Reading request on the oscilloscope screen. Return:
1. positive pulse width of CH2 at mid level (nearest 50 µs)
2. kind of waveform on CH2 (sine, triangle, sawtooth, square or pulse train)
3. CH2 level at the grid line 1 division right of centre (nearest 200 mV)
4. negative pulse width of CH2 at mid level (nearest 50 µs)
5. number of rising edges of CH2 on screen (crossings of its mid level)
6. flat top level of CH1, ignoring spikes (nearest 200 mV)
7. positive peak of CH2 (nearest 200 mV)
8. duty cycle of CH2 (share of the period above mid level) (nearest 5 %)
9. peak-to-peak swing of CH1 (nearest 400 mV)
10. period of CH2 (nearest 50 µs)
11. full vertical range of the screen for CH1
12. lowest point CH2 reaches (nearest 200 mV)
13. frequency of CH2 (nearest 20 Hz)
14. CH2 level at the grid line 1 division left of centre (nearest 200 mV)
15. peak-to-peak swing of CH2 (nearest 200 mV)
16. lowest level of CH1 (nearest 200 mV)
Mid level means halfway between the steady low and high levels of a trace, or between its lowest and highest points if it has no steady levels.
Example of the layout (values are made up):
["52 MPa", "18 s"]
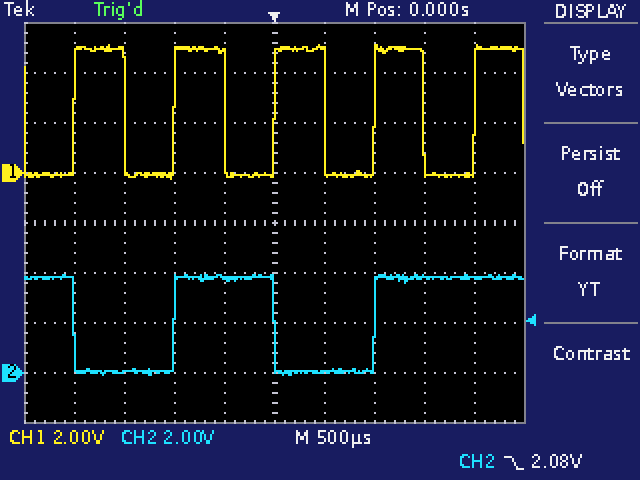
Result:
["1.00 ms", "square", "0.0 V", "1.00 ms", "2", "5.0 V", "4.0 V", "50 %", "5.2 V", "2.00 ms", "16 V", "0.0 V", "500 Hz", "3.8 V", "4.0 V", "-200 mV"]
